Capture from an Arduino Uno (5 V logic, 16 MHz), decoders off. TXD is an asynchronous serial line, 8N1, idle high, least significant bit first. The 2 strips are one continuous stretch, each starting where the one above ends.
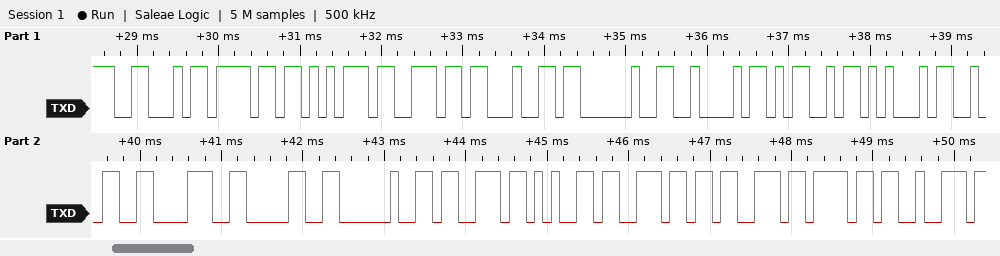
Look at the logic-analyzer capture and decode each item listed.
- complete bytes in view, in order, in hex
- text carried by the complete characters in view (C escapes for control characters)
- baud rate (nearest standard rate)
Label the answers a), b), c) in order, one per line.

a) 46 6F 75 6E 64 20 42 4D 45 32 38 30 20 73 65 6E 73 6F 72
b) "Found BME280 sensor"
c) 9600 baud
